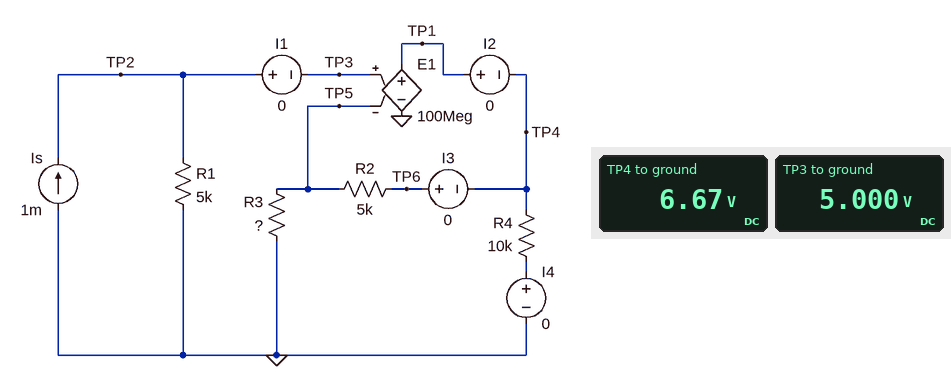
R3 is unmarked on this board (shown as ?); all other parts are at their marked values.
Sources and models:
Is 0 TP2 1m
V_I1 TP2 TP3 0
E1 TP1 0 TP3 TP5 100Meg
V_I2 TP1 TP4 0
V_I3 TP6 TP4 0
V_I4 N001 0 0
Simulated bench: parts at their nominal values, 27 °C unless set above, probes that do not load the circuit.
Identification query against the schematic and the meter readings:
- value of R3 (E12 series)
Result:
15 kΩ
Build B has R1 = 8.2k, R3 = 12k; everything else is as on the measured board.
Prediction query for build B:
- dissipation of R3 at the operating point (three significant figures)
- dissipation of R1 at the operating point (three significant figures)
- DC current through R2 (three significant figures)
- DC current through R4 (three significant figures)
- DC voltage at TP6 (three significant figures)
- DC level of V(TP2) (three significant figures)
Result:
5.60 mW
8.20 mW
683 µA
1.16 mA
11.6 V
8.20 V
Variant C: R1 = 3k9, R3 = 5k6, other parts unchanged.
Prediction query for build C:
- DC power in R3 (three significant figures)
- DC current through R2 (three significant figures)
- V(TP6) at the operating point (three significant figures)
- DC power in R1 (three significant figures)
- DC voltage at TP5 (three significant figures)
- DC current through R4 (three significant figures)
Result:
2.72 mW
696 µA
7.38 V
3.90 mW
3.90 V
738 µA
